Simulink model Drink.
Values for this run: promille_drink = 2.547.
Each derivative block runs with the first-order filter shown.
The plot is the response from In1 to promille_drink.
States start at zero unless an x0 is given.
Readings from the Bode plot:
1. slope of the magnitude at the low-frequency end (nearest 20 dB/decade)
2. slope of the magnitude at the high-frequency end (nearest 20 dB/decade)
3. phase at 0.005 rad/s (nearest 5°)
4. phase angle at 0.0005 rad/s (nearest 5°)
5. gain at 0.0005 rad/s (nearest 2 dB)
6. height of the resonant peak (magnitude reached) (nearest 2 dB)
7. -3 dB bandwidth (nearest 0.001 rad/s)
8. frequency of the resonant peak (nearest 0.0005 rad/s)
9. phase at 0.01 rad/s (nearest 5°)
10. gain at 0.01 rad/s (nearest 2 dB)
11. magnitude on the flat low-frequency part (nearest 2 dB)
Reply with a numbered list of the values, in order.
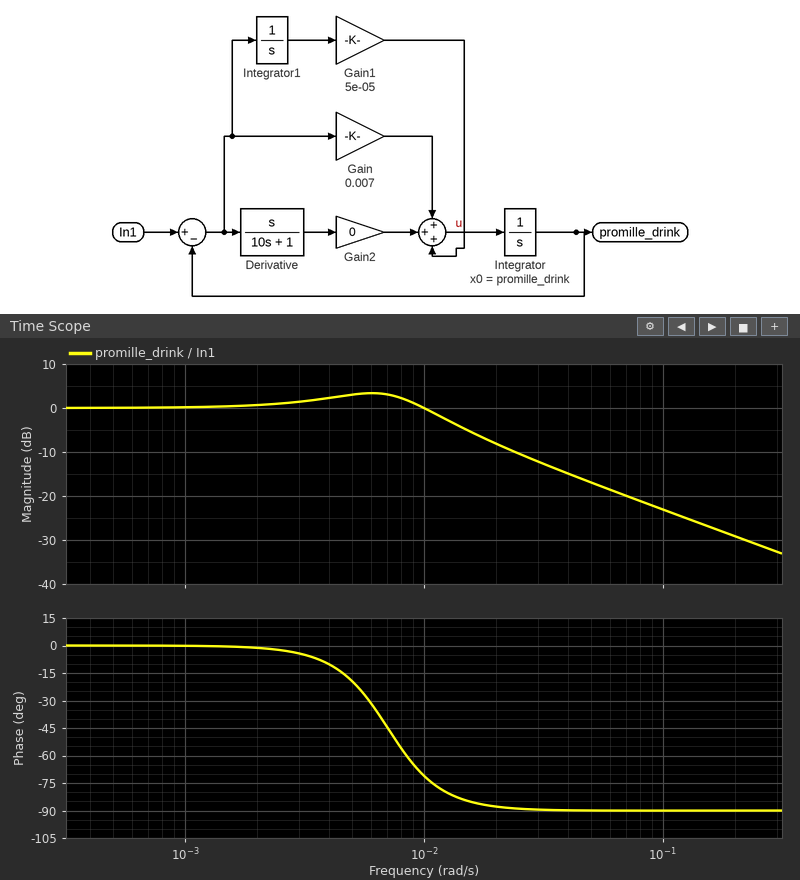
1. 0 dB/decade
2. -20 dB/decade
3. -20°
4. 0°
5. 0 dB
6. 4 dB
7. 0.013 rad/s
8. 0.0060 rad/s
9. -70°
10. 0 dB
11. 0 dB
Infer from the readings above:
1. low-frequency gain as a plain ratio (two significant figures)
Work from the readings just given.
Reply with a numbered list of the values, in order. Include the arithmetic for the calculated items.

1. 10^(0 / 20) = 1.0
